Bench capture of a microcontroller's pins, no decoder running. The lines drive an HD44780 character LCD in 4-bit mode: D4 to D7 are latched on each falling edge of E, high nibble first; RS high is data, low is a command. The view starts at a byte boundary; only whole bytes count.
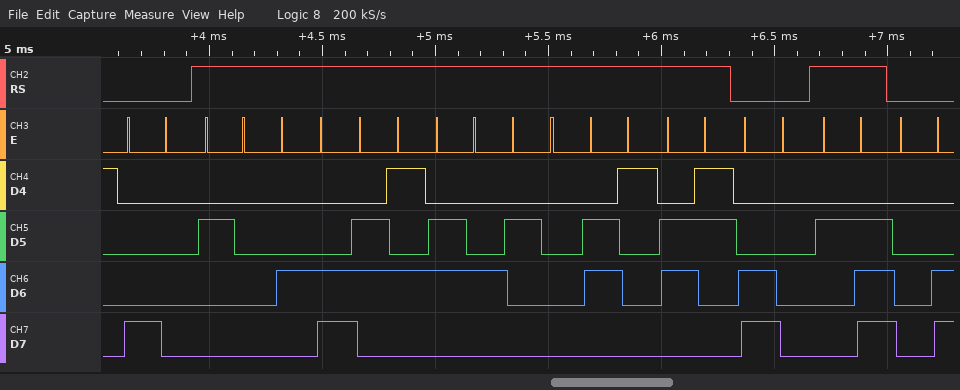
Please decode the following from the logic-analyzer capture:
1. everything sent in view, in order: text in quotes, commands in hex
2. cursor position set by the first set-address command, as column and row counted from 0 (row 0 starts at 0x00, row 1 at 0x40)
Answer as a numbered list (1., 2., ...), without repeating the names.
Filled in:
1. 0x80 " Led ac" 0xC0 "." 0x0C
2. column 0, row 0
